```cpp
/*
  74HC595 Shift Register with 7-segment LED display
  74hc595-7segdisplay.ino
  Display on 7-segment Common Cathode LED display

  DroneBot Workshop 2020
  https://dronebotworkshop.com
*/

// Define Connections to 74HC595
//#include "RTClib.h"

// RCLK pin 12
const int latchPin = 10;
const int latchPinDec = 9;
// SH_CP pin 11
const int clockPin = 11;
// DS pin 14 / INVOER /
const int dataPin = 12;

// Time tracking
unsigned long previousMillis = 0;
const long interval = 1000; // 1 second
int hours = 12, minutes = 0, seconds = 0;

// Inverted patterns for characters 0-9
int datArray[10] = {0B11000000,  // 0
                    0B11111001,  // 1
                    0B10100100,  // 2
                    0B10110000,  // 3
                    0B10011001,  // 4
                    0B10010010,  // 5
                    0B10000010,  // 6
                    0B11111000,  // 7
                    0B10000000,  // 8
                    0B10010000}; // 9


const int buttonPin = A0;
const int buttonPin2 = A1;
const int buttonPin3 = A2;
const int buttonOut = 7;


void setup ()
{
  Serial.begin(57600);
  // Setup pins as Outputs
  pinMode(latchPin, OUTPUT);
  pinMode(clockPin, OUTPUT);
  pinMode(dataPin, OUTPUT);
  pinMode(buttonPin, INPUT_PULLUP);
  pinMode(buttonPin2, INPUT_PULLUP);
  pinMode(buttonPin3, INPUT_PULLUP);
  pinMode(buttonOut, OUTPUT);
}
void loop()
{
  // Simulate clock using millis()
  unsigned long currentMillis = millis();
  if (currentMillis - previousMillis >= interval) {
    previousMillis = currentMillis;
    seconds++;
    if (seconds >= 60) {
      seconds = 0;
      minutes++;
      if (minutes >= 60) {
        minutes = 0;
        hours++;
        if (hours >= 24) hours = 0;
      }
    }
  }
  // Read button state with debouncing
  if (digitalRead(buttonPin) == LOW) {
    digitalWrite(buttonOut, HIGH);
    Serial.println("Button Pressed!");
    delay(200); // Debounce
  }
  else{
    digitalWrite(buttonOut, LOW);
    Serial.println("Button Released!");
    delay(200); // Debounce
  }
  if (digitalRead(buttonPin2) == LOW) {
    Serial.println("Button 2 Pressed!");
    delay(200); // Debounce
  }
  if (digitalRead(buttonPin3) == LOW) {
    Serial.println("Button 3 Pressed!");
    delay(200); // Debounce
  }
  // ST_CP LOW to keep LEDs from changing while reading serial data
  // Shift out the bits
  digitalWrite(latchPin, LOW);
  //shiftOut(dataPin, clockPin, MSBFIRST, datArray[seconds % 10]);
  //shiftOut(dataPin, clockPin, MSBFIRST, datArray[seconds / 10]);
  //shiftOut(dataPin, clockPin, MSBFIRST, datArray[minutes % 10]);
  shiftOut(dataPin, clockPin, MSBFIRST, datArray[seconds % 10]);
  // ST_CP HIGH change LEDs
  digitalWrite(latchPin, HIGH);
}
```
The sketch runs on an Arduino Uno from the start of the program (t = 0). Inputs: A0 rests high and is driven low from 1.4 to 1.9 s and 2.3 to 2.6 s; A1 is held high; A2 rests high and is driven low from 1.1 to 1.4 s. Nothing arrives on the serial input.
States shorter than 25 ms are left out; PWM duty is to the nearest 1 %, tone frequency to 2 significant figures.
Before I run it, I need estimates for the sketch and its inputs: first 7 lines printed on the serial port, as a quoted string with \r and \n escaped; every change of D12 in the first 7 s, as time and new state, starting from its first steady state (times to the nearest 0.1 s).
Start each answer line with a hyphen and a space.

- "Button Released!\r\nButton Released!\r\nButton Released!\r\nButton Released!\r\nButton Released!\r\nButton Released!\r\nButton 3 Pressed!\r\n"
- 0 s low; 1.4 s high; 2.2 s low; 4.2 s high; 5.2 s low
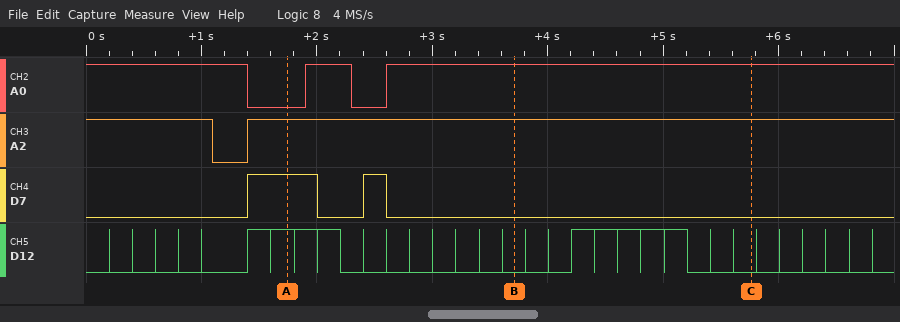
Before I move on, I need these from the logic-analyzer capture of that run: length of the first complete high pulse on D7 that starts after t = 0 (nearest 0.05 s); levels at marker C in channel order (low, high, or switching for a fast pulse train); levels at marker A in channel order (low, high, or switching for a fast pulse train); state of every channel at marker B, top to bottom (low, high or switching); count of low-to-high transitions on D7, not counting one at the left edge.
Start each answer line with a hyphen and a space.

- 0.60 s
- A0 high, A2 high, D7 low, D12 low
- A0 low, A2 high, D7 high, D12 high
- A0 high, A2 high, D7 low, D12 low
- 2
